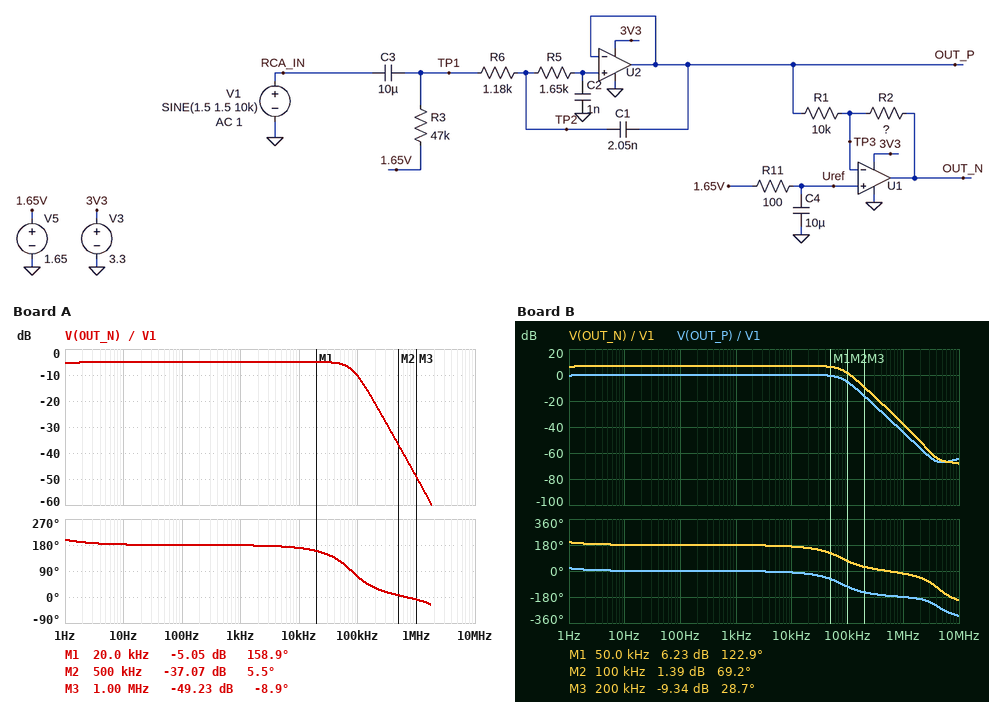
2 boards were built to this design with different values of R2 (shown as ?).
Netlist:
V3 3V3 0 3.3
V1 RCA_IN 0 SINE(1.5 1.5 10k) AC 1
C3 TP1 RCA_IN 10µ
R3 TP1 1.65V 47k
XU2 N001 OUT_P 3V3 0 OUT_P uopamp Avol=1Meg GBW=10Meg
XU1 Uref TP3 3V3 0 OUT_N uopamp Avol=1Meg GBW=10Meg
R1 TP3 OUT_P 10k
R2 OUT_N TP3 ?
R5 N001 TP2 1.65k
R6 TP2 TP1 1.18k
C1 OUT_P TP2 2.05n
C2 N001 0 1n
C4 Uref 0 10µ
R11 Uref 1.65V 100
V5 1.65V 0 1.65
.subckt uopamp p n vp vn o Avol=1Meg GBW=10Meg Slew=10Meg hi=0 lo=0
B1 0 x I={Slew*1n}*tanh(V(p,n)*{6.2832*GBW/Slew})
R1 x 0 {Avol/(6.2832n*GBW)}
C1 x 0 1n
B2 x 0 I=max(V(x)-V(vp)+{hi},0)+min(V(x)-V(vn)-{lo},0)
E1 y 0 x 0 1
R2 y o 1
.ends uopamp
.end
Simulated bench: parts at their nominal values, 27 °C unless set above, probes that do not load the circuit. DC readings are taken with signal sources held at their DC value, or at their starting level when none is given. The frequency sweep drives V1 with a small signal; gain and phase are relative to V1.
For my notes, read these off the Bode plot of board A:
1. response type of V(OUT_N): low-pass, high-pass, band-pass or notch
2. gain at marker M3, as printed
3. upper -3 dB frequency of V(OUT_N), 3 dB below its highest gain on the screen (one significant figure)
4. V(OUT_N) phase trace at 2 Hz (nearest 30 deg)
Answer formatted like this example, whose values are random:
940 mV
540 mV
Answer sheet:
low-pass
-49.23 dB
80 kHz
180 deg
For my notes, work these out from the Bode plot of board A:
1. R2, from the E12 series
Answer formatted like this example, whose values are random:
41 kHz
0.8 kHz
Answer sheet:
5.6 kΩ
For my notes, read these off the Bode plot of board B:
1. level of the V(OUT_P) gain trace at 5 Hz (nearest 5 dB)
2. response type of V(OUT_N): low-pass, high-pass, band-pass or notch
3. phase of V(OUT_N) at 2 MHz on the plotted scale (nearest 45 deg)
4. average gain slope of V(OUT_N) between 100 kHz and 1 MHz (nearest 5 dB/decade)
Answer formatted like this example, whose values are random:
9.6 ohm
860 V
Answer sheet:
0 dB
low-pass
-45 deg
-40 dB/decade
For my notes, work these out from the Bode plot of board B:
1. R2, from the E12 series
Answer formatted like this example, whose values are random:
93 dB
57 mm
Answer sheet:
22 kΩ
